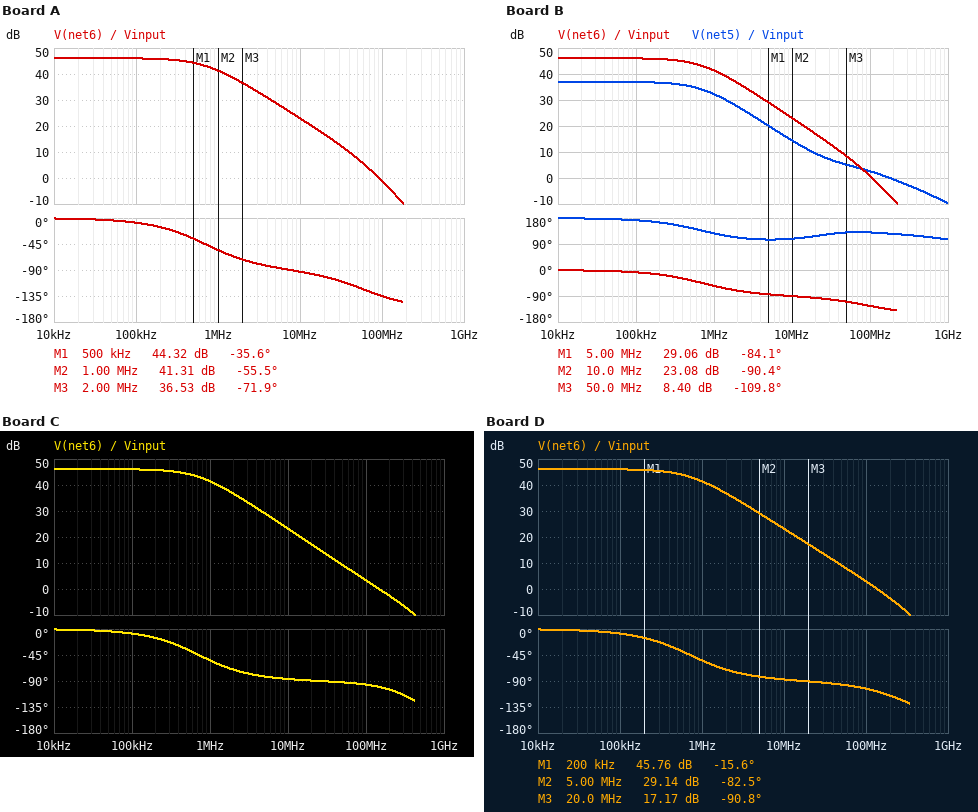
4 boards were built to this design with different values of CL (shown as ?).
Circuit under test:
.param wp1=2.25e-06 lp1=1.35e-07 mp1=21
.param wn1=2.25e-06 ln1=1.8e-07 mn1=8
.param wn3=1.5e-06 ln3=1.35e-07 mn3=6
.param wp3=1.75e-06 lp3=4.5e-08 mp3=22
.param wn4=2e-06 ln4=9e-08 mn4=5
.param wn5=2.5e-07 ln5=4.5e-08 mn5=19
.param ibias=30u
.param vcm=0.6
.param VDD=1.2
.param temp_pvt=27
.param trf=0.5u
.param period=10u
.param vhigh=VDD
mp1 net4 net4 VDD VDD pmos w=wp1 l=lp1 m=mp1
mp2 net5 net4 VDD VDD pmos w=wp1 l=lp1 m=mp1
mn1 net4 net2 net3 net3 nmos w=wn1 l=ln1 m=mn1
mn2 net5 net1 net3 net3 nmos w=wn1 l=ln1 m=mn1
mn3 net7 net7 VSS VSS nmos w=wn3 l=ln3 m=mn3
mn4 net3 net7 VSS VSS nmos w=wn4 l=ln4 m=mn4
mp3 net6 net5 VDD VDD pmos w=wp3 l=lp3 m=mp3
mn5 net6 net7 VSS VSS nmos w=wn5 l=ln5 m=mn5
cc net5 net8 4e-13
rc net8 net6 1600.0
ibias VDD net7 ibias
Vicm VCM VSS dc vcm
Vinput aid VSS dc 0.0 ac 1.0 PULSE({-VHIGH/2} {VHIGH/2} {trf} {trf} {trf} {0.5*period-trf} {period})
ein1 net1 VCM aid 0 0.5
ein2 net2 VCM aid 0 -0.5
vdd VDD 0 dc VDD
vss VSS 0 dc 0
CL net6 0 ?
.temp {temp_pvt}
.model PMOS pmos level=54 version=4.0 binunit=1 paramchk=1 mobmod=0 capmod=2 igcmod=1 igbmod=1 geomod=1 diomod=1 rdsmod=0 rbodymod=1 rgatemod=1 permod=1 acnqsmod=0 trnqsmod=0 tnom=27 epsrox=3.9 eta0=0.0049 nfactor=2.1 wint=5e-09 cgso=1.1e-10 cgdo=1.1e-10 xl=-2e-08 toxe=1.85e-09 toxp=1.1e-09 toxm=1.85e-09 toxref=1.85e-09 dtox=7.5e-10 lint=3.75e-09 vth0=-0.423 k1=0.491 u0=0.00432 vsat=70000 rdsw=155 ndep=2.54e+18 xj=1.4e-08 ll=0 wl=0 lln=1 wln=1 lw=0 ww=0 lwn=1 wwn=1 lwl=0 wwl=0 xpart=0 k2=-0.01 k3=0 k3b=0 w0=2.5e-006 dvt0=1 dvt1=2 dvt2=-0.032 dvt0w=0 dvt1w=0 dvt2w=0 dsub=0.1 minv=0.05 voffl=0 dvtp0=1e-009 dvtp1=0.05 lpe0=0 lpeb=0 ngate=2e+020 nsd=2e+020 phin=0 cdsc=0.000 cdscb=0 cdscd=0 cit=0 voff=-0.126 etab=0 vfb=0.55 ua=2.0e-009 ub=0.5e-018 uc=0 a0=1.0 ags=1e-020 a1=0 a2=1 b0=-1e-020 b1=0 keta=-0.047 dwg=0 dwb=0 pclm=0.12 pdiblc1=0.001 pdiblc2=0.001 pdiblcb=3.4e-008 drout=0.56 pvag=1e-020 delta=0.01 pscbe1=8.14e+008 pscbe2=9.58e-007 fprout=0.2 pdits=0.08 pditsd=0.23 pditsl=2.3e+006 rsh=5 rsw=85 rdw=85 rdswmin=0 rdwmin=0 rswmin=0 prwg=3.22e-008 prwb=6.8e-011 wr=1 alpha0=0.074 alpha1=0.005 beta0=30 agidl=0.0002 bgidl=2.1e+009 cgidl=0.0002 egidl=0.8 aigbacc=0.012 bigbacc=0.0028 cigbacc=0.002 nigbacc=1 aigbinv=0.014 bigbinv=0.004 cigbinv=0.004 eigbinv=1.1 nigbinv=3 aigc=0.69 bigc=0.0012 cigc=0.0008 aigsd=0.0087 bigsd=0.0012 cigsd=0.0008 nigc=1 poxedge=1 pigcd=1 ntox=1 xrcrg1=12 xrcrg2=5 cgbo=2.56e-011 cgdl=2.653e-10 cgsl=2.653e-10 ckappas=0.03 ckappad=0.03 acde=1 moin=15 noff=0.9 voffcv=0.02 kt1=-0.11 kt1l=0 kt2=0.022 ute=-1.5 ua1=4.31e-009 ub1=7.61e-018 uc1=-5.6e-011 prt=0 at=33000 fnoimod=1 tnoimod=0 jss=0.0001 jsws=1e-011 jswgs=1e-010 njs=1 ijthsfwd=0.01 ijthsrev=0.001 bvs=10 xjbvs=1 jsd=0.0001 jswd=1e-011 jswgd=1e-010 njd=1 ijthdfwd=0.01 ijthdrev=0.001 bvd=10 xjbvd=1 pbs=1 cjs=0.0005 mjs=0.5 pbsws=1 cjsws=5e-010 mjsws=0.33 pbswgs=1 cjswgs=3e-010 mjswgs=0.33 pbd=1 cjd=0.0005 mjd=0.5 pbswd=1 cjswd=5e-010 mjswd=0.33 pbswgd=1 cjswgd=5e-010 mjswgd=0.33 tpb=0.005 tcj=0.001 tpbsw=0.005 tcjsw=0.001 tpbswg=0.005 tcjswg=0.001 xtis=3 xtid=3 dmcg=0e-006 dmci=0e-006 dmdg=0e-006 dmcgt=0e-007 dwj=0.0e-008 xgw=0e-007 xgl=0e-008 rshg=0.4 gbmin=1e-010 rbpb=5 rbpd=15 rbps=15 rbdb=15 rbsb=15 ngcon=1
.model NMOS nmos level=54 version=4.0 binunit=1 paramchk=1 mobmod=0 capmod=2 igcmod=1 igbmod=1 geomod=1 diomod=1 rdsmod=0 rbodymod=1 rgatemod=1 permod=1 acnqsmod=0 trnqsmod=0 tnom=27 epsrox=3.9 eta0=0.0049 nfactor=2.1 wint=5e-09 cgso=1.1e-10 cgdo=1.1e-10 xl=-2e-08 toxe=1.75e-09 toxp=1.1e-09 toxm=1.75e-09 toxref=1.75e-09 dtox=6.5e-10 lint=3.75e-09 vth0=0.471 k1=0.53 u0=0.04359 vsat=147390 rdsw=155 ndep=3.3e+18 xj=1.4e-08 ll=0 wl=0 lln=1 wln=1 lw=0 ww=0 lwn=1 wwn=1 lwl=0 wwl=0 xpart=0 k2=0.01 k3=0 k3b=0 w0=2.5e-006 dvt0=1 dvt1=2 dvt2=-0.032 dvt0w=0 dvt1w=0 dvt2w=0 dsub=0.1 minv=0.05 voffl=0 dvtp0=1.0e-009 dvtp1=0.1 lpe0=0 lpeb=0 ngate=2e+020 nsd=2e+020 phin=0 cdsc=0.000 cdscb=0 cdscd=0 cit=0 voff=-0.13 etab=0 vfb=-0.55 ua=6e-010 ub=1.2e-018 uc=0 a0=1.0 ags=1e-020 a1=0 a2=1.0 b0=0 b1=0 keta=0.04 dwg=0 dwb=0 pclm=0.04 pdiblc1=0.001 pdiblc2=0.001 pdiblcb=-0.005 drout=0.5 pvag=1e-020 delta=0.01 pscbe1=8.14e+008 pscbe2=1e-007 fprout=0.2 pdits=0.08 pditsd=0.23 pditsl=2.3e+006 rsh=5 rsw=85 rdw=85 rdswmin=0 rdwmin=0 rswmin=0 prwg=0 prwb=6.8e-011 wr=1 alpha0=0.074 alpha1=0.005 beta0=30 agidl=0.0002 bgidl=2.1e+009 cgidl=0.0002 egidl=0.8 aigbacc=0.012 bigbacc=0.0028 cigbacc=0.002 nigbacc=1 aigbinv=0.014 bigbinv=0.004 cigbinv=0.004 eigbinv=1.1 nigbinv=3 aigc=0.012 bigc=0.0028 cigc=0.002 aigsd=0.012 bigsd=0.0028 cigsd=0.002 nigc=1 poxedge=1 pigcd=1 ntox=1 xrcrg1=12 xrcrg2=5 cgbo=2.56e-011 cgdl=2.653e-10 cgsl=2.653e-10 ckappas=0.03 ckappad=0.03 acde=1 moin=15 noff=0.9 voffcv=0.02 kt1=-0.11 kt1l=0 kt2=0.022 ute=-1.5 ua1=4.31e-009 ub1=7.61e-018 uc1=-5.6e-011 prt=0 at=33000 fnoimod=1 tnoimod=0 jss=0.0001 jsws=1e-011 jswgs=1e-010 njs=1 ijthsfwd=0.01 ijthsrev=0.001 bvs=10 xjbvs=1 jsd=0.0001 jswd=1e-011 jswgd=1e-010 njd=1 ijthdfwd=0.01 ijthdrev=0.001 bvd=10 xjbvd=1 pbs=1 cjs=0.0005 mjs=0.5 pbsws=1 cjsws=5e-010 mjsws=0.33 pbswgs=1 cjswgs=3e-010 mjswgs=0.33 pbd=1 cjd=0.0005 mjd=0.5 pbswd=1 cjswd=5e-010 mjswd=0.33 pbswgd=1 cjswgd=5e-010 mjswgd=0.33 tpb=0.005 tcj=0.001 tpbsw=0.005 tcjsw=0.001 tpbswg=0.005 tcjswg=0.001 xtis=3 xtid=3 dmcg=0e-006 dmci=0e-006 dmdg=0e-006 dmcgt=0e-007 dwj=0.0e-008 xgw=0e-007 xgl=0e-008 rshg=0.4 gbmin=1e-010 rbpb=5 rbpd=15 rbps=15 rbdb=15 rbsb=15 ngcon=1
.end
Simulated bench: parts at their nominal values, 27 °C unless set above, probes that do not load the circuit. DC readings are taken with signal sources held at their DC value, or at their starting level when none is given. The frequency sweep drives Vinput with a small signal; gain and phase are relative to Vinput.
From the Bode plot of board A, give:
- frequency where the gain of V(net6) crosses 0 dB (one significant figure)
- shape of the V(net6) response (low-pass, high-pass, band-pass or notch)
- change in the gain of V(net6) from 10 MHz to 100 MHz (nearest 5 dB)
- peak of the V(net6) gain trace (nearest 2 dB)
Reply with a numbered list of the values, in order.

1. 90 MHz
2. low-pass
3. -25 dB
4. 46 dB
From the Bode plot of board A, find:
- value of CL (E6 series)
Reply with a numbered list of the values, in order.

1. 22 pF
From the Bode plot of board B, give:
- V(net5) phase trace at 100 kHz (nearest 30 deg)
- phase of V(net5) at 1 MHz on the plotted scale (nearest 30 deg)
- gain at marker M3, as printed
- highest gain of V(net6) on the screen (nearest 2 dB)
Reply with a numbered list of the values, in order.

1. 180 deg
2. 120 deg
3. 8.40 dB
4. 46 dB
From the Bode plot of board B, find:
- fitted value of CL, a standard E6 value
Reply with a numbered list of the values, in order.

1. 15 pF
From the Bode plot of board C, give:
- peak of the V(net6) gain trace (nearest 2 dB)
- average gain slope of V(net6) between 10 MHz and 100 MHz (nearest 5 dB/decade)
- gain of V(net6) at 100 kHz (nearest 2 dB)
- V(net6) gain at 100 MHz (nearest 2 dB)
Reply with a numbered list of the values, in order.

1. 46 dB
2. -20 dB/decade
3. 46 dB
4. 4 dB
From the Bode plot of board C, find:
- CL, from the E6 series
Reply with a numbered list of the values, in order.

1. 4.7 pF
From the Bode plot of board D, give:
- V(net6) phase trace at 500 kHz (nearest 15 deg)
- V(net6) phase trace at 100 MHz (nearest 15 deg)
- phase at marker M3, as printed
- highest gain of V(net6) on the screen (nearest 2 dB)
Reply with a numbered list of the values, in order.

1. -30 deg
2. -105 deg
3. -90.8 deg
4. 46 dB
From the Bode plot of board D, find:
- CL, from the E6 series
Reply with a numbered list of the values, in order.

1. 6.8 pF
